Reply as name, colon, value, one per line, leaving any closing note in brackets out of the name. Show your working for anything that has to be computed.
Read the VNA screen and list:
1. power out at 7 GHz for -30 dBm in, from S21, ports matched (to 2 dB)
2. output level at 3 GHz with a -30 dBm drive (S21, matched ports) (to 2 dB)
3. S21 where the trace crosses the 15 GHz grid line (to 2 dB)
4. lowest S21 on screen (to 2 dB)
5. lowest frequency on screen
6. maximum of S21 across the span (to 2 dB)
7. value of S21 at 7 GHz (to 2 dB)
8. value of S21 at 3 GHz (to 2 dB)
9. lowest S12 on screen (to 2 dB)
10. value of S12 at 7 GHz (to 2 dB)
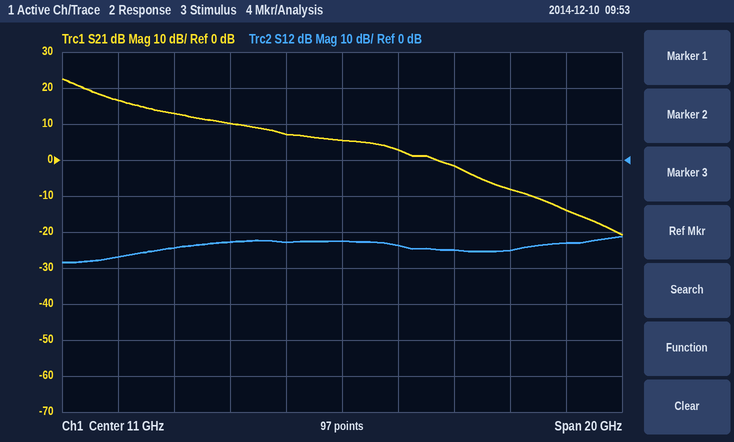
power out at 7 GHz for -30 dBm in, from S21, ports matched: -30 dBm + (10 dB) = -20 dBm
output level at 3 GHz with a -30 dBm drive (S21, matched ports): -30 dBm + (16 dB) = -14 dBm
S21 where the trace crosses the 15 GHz grid line: -2 dB
lowest S21 on screen: -20 dB
lowest frequency on screen: 1 GHz
maximum of S21 across the span: 22 dB
value of S21 at 7 GHz: 10 dB
value of S21 at 3 GHz: 16 dB
lowest S12 on screen: -28 dB
value of S12 at 7 GHz: -22 dB
